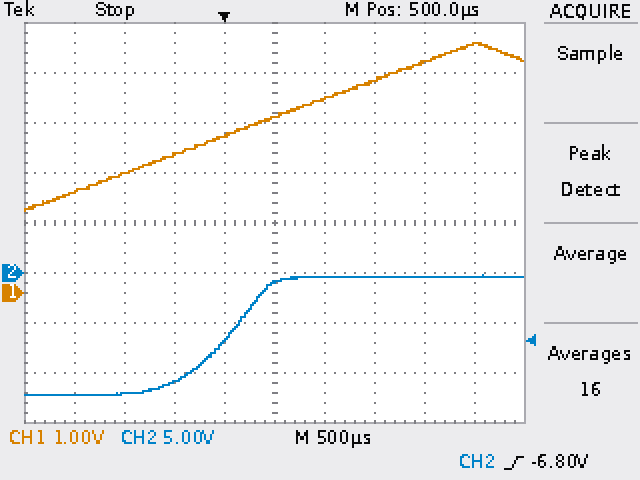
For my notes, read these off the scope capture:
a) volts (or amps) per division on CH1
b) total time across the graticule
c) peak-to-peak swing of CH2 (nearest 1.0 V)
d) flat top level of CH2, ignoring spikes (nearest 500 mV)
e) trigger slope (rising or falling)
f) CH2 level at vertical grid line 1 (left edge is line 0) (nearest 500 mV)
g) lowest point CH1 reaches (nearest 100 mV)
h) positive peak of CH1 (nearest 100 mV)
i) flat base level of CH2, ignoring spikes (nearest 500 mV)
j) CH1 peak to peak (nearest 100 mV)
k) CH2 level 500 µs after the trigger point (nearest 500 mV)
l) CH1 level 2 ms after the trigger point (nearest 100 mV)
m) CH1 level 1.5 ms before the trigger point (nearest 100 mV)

1 V
5 ms
12.0 V
-500 mV
rising
-12.0 V
1.6 V
5.0 V
-12.0 V
3.4 V
-1.0 V
4.6 V
2.0 V
